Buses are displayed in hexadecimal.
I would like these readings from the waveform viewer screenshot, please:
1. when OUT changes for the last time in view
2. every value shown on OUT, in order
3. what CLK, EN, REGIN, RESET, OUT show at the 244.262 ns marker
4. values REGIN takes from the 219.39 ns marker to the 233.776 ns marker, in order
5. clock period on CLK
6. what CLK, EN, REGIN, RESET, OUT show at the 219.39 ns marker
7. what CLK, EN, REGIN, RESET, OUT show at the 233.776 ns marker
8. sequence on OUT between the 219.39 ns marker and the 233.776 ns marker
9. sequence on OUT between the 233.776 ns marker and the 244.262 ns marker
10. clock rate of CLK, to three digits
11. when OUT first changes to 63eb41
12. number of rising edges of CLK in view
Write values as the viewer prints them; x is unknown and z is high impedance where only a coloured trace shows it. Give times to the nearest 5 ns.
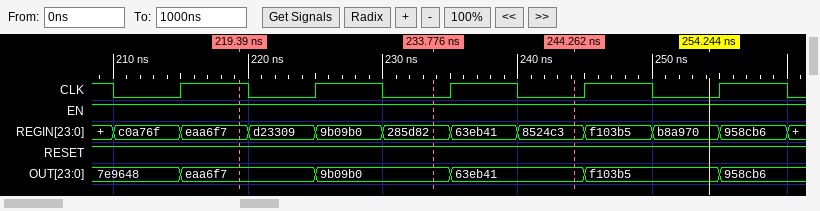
255 ns
7e9648, eaa6f7, 9b09b0, 63eb41, f103b5, 958cb6
CLK=0, EN=1, REGIN=8524c3, RESET=1, OUT=63eb41
eaa6f7, d23309, 9b09b0, 285d82
10 ns
CLK=1, EN=1, REGIN=eaa6f7, RESET=1, OUT=eaa6f7
CLK=0, EN=1, REGIN=285d82, RESET=1, OUT=9b09b0
eaa6f7, 9b09b0
9b09b0, 63eb41
100 MHz
235 ns
5
